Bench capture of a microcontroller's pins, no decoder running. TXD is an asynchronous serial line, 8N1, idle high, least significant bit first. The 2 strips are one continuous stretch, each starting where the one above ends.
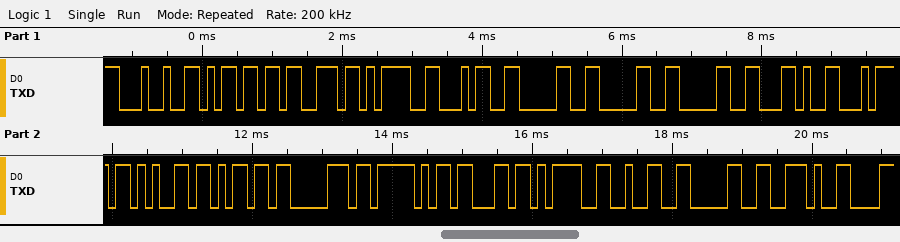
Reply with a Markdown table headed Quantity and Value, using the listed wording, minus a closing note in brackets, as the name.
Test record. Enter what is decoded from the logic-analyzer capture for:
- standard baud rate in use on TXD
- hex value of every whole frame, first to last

| Quantity | Value |
|---|---|
| standard baud rate in use on TXD | 9600 baud |
| hex value of every whole frame, first to last | 0x24 0x6D 0x73 0x3D 0x34 0x30 0x30 0x30 0x2C 0x74 0x65 0x6D 0x70 0x5F 0x63 0x3D 0x32 0x30 0x2E |
